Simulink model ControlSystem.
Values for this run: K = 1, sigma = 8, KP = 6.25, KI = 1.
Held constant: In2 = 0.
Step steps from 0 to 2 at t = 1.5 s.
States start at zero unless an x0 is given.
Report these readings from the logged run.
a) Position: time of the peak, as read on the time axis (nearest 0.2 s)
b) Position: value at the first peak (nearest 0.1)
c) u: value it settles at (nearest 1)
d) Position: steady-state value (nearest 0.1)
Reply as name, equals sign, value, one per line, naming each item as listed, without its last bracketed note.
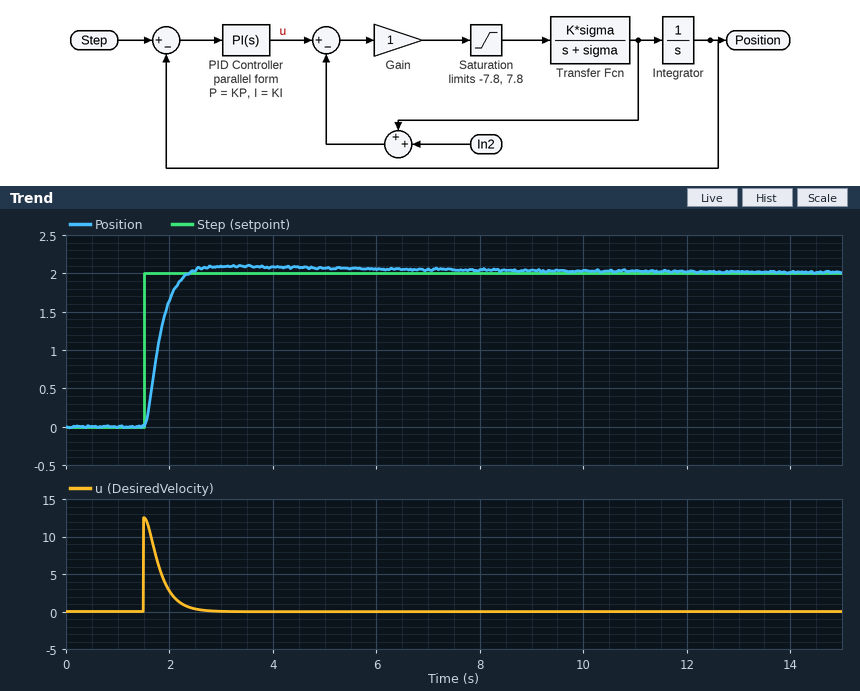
Position: time of the peak, as read on the time axis = 3.2 s
Position: value at the first peak = 2.1
u: value it settles at = 0
Position: steady-state value = 2.0
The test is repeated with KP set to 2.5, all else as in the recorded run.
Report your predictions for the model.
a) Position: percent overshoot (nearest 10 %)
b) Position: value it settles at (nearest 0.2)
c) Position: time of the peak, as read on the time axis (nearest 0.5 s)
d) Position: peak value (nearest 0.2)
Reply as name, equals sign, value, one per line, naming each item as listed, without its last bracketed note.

Position: percent overshoot = 20 %
Position: value it settles at = 2.0
Position: time of the peak, as read on the time axis = 4.5 s
Position: peak value = 2.4
